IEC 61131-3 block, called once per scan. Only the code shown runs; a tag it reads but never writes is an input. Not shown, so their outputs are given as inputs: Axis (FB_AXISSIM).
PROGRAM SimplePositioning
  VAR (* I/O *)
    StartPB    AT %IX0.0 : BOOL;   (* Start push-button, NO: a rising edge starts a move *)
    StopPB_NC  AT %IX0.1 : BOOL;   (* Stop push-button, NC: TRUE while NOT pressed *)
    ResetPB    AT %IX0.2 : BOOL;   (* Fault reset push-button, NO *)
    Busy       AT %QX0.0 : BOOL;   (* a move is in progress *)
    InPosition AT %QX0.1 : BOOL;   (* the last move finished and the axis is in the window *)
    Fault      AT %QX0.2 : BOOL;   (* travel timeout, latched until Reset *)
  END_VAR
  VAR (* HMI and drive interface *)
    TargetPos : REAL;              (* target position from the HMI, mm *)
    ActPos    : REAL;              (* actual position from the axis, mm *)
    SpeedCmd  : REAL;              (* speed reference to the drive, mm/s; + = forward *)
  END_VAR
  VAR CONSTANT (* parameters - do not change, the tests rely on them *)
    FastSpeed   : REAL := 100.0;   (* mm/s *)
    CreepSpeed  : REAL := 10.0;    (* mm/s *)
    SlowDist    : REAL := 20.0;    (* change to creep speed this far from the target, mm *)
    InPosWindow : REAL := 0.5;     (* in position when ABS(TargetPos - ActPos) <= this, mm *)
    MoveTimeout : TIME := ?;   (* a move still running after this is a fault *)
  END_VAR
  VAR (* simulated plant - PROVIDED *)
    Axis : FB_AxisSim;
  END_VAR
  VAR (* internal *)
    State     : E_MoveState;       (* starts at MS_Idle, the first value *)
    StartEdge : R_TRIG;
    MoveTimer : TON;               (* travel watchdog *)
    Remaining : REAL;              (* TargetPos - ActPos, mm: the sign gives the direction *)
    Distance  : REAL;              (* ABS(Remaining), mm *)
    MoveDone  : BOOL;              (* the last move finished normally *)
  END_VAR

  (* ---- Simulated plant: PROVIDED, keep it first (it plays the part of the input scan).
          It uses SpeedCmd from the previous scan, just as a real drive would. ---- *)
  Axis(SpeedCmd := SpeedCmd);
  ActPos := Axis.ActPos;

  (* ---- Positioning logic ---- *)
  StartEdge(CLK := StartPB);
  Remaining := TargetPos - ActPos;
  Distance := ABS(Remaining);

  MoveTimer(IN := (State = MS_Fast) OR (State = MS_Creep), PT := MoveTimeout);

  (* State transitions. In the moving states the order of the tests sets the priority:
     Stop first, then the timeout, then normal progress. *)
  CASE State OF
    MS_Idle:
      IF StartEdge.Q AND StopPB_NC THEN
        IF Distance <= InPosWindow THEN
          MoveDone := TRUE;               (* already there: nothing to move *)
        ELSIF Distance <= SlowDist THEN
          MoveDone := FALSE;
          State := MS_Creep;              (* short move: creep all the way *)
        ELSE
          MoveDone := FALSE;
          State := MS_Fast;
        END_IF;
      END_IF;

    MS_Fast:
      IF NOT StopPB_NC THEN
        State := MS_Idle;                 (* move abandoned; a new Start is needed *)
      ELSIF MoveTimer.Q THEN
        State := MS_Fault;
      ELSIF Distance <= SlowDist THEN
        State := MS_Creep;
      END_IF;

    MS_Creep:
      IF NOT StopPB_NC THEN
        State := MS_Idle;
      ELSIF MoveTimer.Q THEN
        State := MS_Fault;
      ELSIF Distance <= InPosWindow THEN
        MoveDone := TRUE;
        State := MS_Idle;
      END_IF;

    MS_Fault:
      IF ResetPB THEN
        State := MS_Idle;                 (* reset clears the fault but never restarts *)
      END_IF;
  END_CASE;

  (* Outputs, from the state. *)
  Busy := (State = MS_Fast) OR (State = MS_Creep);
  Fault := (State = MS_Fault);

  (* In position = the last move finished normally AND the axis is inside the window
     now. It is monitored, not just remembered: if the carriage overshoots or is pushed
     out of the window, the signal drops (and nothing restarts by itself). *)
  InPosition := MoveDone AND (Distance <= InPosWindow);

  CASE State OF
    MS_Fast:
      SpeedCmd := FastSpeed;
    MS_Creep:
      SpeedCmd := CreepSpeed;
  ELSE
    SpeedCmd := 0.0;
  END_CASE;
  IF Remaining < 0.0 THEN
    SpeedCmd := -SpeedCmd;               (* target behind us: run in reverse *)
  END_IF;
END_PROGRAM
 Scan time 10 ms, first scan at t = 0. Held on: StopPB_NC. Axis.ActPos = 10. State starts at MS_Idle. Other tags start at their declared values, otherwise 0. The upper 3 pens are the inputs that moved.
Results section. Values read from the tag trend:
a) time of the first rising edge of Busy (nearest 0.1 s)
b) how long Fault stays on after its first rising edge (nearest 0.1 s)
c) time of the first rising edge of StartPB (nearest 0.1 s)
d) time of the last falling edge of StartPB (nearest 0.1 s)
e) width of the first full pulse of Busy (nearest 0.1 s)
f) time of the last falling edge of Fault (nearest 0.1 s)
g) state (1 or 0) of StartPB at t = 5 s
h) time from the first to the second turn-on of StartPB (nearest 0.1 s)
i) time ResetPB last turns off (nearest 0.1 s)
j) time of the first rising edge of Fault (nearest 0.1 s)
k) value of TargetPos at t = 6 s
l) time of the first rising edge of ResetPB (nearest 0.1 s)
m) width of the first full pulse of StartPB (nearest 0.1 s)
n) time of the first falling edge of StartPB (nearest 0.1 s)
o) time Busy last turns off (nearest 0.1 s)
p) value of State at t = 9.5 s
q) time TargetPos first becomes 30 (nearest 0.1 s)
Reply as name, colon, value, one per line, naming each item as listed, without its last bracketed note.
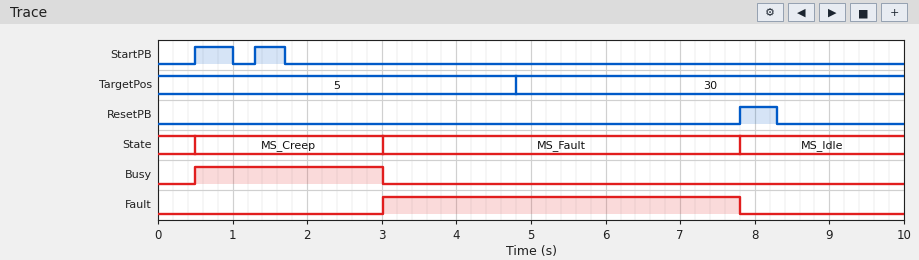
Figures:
time of the first rising edge of Busy: 0.5 s
how long Fault stays on after its first rising edge: 4.8 s
time of the first rising edge of StartPB: 0.5 s
time of the last falling edge of StartPB: 1.7 s
width of the first full pulse of Busy: 2.5 s
time of the last falling edge of Fault: 7.8 s
state (1 or 0) of StartPB at t = 5 s: 0
time from the first to the second turn-on of StartPB: 0.8 s
time ResetPB last turns off: 8.3 s
time of the first rising edge of Fault: 3.0 s
value of TargetPos at t = 6 s: 30
time of the first rising edge of ResetPB: 7.8 s
width of the first full pulse of StartPB: 0.5 s
time of the first falling edge of StartPB: 1.0 s
time Busy last turns off: 3.0 s
value of State at t = 9.5 s: MS_Idle
time TargetPos first becomes 30: 4.8 s
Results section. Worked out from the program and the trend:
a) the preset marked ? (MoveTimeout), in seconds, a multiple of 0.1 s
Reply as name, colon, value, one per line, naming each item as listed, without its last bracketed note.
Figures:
the preset marked ? (MoveTimeout), in seconds, a multiple of 0.1 s: 2.5 s
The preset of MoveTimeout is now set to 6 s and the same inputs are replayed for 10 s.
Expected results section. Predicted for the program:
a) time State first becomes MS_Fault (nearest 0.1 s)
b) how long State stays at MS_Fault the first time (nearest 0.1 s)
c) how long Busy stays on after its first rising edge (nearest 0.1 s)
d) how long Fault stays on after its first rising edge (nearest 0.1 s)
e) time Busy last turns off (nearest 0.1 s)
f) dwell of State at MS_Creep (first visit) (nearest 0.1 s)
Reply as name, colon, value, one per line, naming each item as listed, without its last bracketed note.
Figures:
time State first becomes MS_Fault: 6.5 s
how long State stays at MS_Fault the first time: 1.3 s
how long Busy stays on after its first rising edge: 6.0 s
how long Fault stays on after its first rising edge: 1.3 s
time Busy last turns off: 6.5 s
dwell of State at MS_Creep (first visit): 6.0 s
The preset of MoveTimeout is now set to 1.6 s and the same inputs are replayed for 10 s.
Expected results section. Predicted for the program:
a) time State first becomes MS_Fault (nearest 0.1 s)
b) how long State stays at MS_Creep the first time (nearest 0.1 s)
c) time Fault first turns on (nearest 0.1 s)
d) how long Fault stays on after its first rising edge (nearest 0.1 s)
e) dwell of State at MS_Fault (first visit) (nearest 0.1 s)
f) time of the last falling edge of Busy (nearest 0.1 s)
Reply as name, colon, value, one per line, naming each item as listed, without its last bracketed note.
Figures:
time State first becomes MS_Fault: 2.1 s
how long State stays at MS_Creep the first time: 1.6 s
time Fault first turns on: 2.1 s
how long Fault stays on after its first rising edge: 5.7 s
dwell of State at MS_Fault (first visit): 5.7 s
time of the last falling edge of Busy: 2.1 s
